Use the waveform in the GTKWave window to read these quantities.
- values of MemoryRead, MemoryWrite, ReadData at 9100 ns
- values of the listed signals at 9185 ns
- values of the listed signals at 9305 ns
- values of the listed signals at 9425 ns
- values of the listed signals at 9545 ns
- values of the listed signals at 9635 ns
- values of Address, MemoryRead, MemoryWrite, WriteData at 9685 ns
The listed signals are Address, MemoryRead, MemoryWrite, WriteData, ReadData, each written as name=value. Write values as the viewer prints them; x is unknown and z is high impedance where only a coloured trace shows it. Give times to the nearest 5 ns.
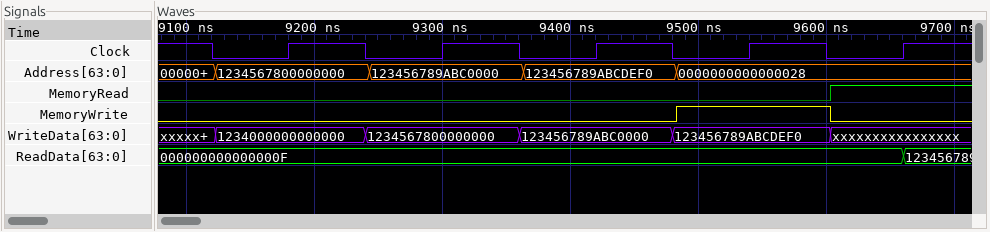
MemoryRead=0, MemoryWrite=0, ReadData=000000000000000F
Address=1234567800000000, MemoryRead=0, MemoryWrite=0, WriteData=1234000000000000, ReadData=000000000000000F
Address=123456789ABC0000, MemoryRead=0, MemoryWrite=0, WriteData=1234567800000000, ReadData=000000000000000F
Address=123456789ABCDEF0, MemoryRead=0, MemoryWrite=0, WriteData=123456789ABC0000, ReadData=000000000000000F
Address=0000000000000028, MemoryRead=0, MemoryWrite=1, WriteData=123456789ABCDEF0, ReadData=000000000000000F
Address=0000000000000028, MemoryRead=1, MemoryWrite=0, WriteData=xxxxxxxxxxxxxxxx, ReadData=000000000000000F
Address=0000000000000028, MemoryRead=1, MemoryWrite=0, WriteData=xxxxxxxxxxxxxxxx
